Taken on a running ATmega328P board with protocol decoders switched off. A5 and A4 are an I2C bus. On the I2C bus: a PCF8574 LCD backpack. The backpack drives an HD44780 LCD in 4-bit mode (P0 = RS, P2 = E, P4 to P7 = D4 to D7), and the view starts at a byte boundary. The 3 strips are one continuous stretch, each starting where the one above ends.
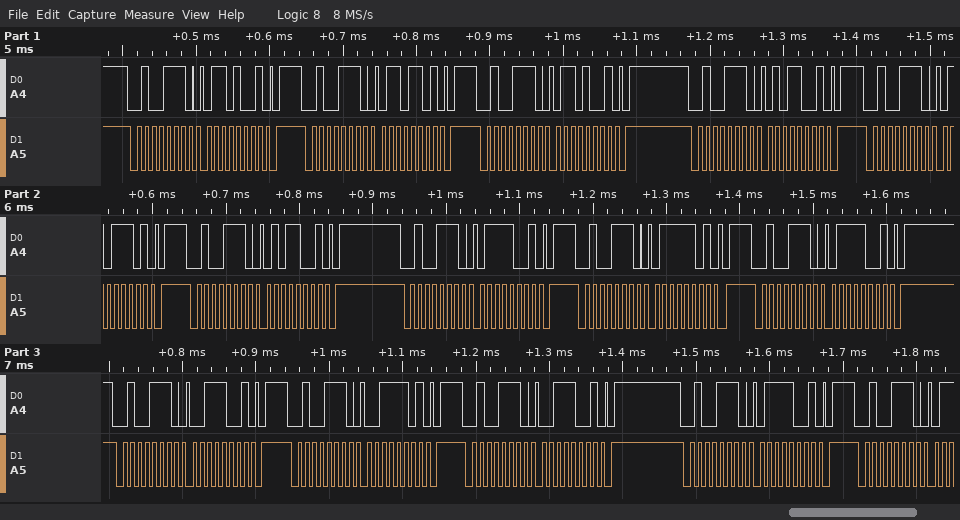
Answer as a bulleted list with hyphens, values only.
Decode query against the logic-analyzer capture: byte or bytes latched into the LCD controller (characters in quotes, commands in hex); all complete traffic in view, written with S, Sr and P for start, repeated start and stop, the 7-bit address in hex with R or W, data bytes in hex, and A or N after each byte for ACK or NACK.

- 'e' 's'
- S 27W A 69 A P S 27W A 6D A P S 27W A 69 A P S 27W A 59 A P S 27W A 5D A P S 27W A 59 A P S 27W A 79 A P S 27W A 7D A P S 27W A 79 A P S 27W A 39 A P S 27W A 3D A P S 27W A 39 A P S 27W A 79 A P S 27W A
